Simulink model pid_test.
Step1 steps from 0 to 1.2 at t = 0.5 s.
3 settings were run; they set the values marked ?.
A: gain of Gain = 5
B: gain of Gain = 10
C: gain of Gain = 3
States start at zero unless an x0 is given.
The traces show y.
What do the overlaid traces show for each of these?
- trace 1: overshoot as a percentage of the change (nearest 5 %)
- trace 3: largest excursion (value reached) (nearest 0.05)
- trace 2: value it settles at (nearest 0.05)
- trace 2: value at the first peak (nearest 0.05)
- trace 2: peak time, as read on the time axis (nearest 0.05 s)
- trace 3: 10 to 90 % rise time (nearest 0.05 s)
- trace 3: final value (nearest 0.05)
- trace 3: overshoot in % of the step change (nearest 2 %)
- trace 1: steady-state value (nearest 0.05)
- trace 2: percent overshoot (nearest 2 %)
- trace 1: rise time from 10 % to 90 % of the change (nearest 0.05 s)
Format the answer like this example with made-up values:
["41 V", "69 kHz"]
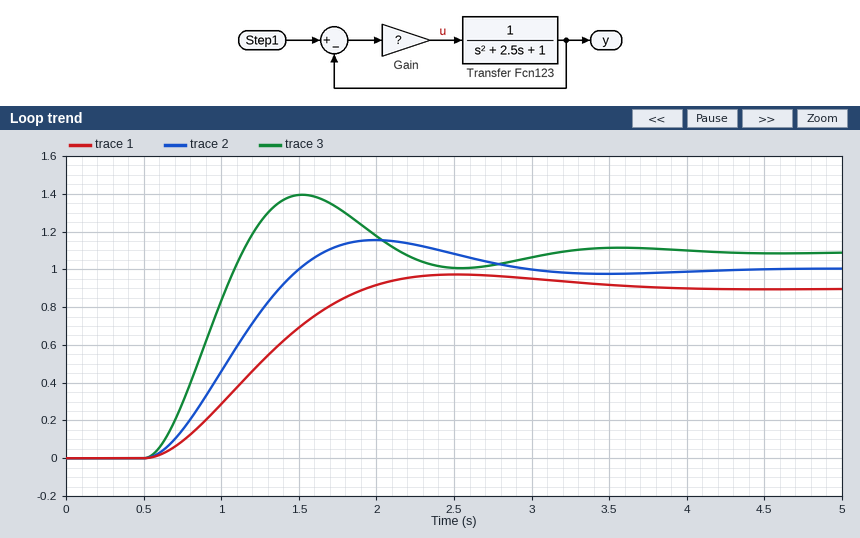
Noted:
["10 %", "1.40", "1.00", "1.15", "2.00 s", "0.45 s", "1.10", "28 %", "0.90", "16 %", "0.95 s"]
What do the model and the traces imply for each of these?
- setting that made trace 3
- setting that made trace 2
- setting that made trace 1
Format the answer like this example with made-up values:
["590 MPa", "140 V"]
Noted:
["B", "A", "C"]
